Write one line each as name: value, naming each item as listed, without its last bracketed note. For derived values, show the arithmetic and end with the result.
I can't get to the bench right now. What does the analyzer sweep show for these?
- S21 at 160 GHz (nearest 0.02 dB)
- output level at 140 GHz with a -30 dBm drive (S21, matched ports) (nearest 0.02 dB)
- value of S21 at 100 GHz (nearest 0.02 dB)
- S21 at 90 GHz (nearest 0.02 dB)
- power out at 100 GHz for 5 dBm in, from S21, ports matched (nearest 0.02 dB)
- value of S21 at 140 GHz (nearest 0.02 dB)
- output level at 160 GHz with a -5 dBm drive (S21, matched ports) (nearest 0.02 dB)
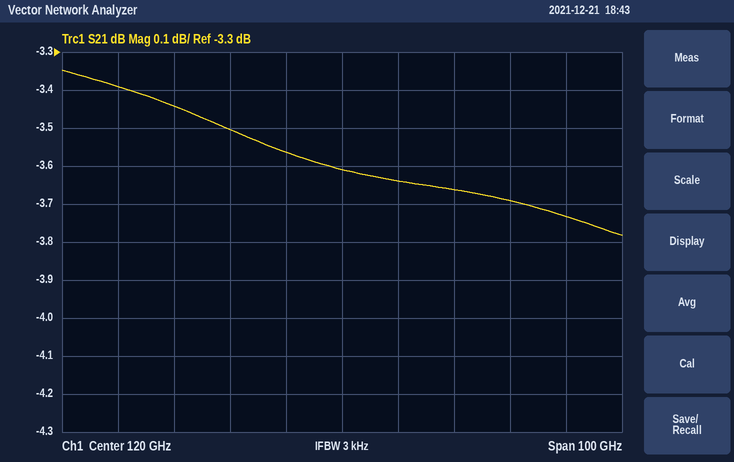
S21 at 160 GHz: -3.74 dB
output level at 140 GHz with a -30 dBm drive (S21, matched ports): -30 dBm + (-3.66 dB) = -33.66 dBm
value of S21 at 100 GHz: -3.50 dB
S21 at 90 GHz: -3.44 dB
power out at 100 GHz for 5 dBm in, from S21, ports matched: 5 dBm + (-3.50 dB) = 1.50 dBm
value of S21 at 140 GHz: -3.66 dB
output level at 160 GHz with a -5 dBm drive (S21, matched ports): -5 dBm + (-3.74 dB) = -8.74 dBm
